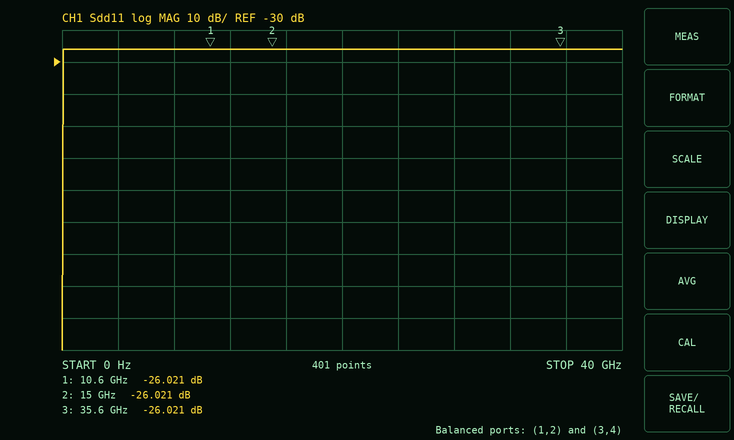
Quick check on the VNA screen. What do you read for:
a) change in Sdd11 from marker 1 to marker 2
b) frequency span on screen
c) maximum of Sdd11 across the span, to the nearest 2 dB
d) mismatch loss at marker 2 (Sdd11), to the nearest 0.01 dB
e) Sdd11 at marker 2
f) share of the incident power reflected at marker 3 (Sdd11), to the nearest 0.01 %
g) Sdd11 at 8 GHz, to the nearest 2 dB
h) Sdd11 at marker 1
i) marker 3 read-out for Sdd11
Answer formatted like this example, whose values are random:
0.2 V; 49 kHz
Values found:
0.000 dB; 40 GHz; -26 dB; 0.01 dB; -26.021 dB; 0.25 %; -26 dB; -26.021 dB; -26.021 dB
